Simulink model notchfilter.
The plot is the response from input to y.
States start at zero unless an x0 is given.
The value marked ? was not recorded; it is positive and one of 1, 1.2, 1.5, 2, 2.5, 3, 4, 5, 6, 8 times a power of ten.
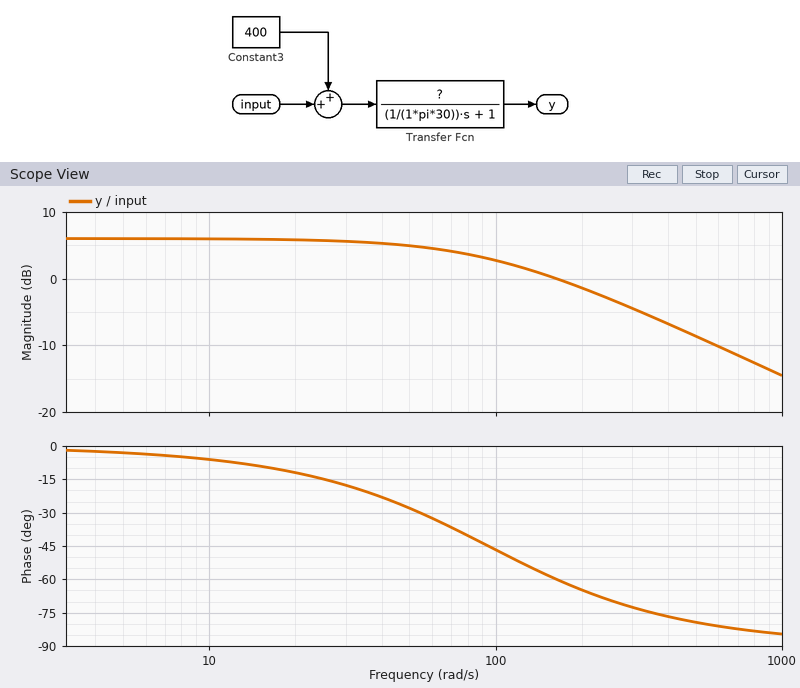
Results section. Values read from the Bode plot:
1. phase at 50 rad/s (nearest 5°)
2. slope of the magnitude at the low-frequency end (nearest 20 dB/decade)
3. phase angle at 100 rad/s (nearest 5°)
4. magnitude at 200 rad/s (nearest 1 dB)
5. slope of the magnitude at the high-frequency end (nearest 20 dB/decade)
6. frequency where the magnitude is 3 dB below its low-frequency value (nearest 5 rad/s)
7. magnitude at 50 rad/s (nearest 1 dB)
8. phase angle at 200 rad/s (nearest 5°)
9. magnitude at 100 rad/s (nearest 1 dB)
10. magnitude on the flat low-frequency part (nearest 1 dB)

-30°
0 dB/decade
-45°
-1 dB
-20 dB/decade
95 rad/s
5 dB
-65°
3 dB
6 dB
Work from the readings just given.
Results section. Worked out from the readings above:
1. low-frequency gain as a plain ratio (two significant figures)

2.0
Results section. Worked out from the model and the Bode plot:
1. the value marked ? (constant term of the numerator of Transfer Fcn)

2
